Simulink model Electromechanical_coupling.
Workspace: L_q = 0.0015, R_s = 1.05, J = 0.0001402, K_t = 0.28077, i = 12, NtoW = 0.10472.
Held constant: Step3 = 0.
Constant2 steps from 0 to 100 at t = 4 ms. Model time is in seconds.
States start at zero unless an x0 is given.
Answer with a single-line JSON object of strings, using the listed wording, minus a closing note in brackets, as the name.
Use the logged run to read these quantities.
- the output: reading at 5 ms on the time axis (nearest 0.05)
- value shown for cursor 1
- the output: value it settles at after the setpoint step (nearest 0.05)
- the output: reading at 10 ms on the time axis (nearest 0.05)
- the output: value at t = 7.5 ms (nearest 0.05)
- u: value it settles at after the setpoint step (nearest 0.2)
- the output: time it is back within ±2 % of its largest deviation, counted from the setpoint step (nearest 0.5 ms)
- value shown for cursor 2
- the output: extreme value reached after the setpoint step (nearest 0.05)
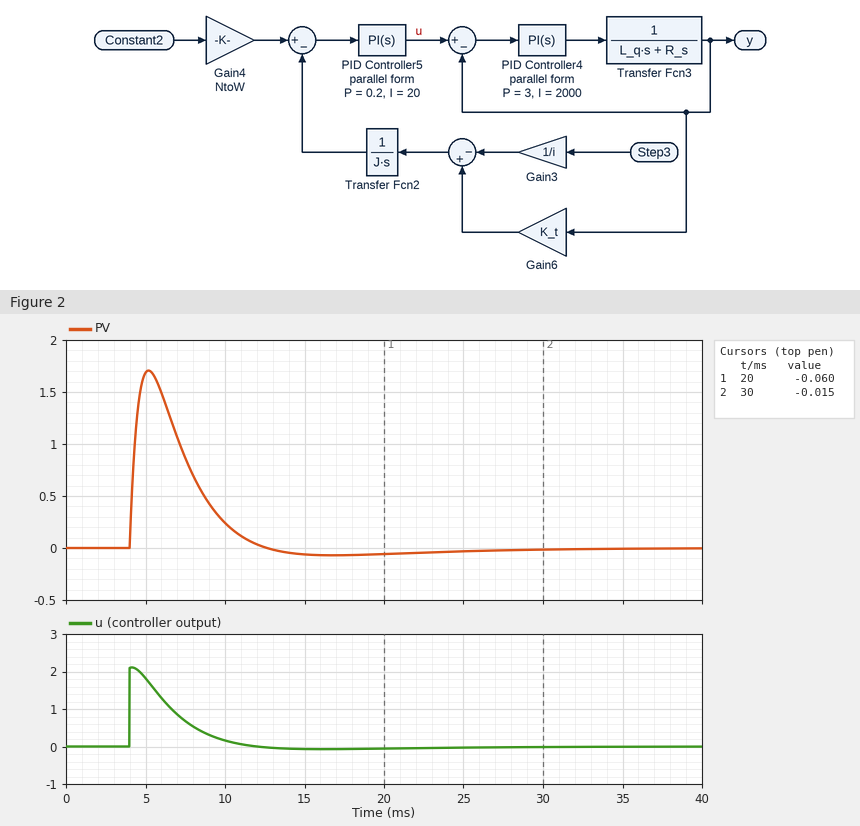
{"the output: reading at 5 ms on the time axis": "1.70", "value shown for cursor 1": "-0.060", "the output: value it settles at after the setpoint step": "0.00", "the output: reading at 10 ms on the time axis": "0.25", "the output: value at t = 7.5 ms": "0.85", "u: value it settles at after the setpoint step": "0.0", "the output: time it is back within ±2 % of its largest deviation, counted from the setpoint step": "20.5 ms", "value shown for cursor 2": "-0.015", "the output: extreme value reached after the setpoint step": "1.70"}
